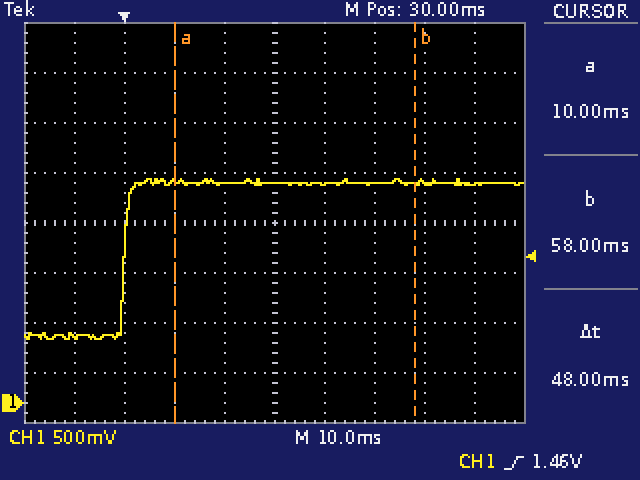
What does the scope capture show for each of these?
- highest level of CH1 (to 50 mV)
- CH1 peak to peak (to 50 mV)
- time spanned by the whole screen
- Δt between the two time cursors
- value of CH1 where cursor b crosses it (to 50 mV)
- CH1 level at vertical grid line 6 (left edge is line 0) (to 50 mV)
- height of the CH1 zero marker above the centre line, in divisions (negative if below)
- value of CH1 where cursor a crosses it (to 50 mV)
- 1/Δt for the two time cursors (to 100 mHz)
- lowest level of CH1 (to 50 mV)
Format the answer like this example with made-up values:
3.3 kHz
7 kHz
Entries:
2.25 V
1.60 V
100 ms
48 ms
2.20 V
2.20 V
-3.6 div
2.20 V
20.8 Hz
650 mV
